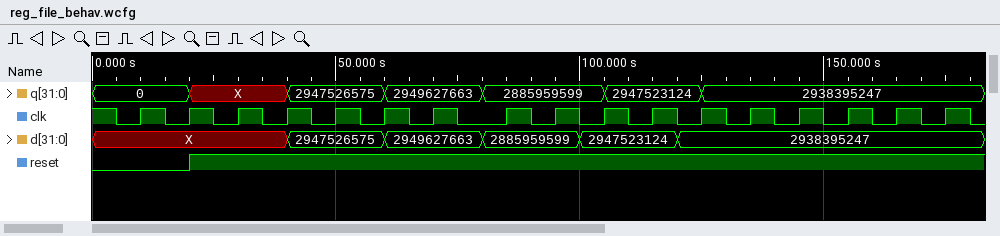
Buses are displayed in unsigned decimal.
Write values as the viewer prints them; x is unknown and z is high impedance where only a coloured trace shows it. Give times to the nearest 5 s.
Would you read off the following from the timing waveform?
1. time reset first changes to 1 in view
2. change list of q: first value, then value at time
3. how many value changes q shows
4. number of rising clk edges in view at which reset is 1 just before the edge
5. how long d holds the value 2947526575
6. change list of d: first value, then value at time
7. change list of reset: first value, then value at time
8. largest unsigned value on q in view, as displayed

20 s
0, X at 20 s, 2947526575 at 40 s, 2949627663 at 60 s, 2885959599 at 80 s, 2947523124 at 105 s, 2938395247 at 125 s
6
15
20 s
X, 2947526575 at 40 s, 2949627663 at 60 s, 2885959599 at 80 s, 2947523124 at 100 s, 2938395247 at 120 s
0, 1 at 20 s
2949627663
